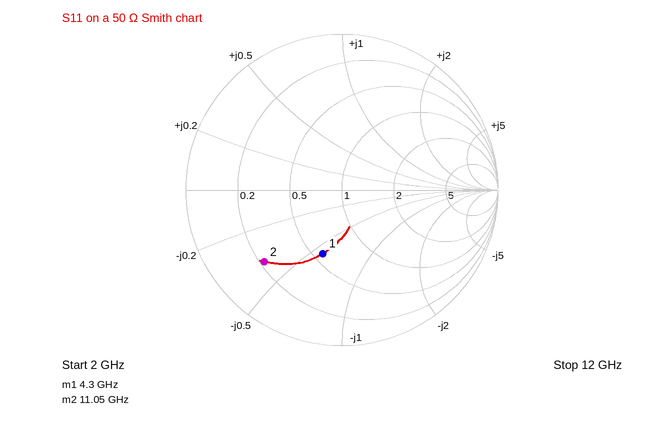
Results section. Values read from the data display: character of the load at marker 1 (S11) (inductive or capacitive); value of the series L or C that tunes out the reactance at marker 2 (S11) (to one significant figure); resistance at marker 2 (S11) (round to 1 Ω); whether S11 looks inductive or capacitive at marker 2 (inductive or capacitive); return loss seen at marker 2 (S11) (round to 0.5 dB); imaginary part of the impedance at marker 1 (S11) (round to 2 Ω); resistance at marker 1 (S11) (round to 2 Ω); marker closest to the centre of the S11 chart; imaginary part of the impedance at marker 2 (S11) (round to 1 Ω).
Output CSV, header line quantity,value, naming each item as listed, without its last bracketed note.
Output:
quantity,value
character of the load at marker 1 (S11),capacitive
value of the series L or C that tunes out the reactance at marker 2 (S11),300 pH
resistance at marker 2 (S11),11 Ω
whether S11 looks inductive or capacitive at marker 2,capacitive
return loss seen at marker 2 (S11),3.5 dB
imaginary part of the impedance at marker 1 (S11),-28 Ω
resistance at marker 1 (S11),28 Ω
marker closest to the centre of the S11 chart,marker 1
imaginary part of the impedance at marker 2 (S11),-19 Ω
